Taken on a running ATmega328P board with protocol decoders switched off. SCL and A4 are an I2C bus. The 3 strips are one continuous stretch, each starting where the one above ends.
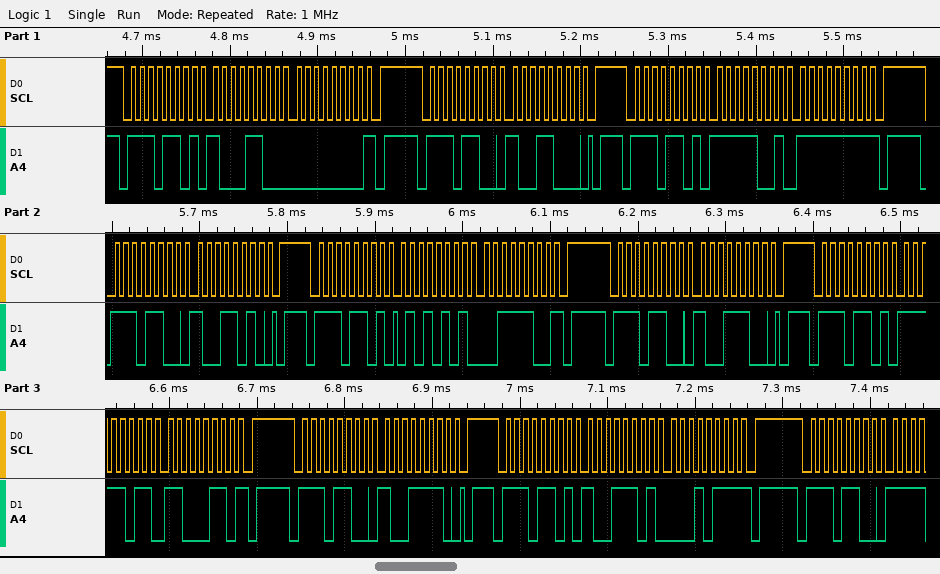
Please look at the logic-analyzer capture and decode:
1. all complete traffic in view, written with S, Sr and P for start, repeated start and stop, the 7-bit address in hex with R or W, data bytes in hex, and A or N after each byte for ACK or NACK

S 76R A 8C A 00 N P S 76W A 98 A P S 76R A F9 A FF N P S 76W A 9A A P S 76R A 55 A 3C N P S 76W A 9C A P S 76R A FB A C6 N P S 76W A 9E A P S 76R A 9D A 17 N P S 76W A
